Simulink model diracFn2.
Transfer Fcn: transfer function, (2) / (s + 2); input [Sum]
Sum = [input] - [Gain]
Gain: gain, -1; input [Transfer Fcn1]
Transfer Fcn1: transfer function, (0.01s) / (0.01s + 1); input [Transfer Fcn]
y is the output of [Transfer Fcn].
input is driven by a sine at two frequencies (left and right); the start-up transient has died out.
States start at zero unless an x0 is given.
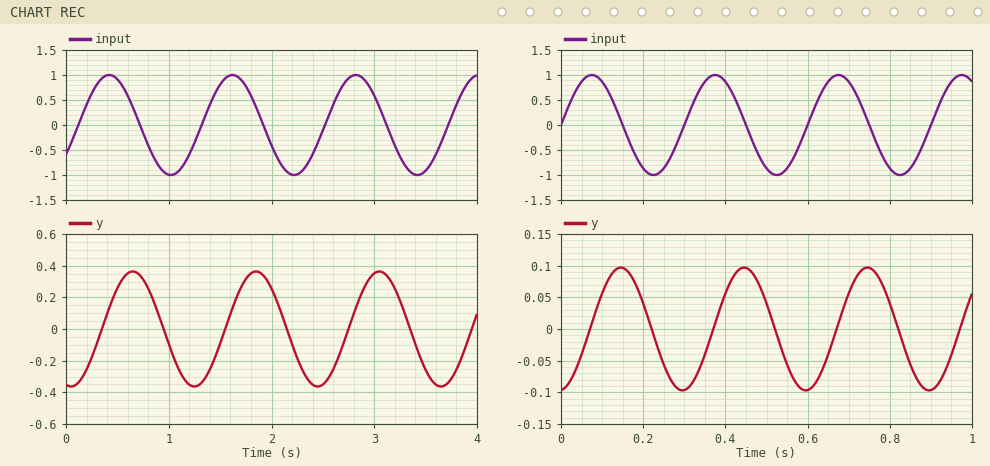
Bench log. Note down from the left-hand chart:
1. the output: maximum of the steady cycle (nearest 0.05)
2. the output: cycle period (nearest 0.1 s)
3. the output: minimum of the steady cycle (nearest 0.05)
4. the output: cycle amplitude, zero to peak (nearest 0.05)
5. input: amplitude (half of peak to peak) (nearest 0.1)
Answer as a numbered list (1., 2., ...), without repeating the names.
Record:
1. 0.35
2. 1.2 s
3. -0.35
4. 0.35
5. 1.0
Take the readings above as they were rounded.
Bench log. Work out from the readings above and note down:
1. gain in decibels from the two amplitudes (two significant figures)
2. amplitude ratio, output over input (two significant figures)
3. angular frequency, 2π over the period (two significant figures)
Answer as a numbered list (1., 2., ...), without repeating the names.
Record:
1. -9.1 dB
2. 0.35
3. 5.2 rad/s
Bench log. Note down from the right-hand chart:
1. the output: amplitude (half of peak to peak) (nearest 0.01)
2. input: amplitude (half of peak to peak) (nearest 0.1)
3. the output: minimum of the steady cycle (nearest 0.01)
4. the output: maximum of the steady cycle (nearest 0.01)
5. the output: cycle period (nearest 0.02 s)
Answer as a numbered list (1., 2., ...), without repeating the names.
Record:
1. 0.10
2. 1.0
3. -0.10
4. 0.10
5. 0.30 s
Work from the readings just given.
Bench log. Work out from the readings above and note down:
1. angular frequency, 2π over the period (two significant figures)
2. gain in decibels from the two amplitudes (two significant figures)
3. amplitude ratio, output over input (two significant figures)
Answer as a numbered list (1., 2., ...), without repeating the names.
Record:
1. 21 rad/s
2. -20 dB
3. 0.10
